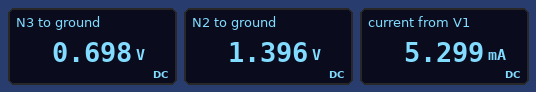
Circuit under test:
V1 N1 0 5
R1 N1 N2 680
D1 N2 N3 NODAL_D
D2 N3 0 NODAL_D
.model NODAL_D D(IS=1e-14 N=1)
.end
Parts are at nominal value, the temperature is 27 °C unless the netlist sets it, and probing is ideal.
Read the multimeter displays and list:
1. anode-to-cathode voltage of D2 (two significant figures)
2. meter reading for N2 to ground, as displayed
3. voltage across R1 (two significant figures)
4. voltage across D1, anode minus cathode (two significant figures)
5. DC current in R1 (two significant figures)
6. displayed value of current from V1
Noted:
700 mV
1.396 V
3.6 V
700 mV
5.3 mA
5.299 mA
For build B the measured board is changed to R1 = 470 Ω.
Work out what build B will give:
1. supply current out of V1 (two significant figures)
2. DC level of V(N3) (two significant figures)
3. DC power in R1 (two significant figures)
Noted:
7.6 mA
710 mV
27 mW
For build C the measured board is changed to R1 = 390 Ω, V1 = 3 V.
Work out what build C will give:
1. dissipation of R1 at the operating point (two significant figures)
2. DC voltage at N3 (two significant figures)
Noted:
6.7 mW
690 mV
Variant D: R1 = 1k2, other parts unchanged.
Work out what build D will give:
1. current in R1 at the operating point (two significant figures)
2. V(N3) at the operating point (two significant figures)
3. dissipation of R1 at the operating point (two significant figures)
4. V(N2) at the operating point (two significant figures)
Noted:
3.0 mA
680 mV
11 mW
1.4 V
